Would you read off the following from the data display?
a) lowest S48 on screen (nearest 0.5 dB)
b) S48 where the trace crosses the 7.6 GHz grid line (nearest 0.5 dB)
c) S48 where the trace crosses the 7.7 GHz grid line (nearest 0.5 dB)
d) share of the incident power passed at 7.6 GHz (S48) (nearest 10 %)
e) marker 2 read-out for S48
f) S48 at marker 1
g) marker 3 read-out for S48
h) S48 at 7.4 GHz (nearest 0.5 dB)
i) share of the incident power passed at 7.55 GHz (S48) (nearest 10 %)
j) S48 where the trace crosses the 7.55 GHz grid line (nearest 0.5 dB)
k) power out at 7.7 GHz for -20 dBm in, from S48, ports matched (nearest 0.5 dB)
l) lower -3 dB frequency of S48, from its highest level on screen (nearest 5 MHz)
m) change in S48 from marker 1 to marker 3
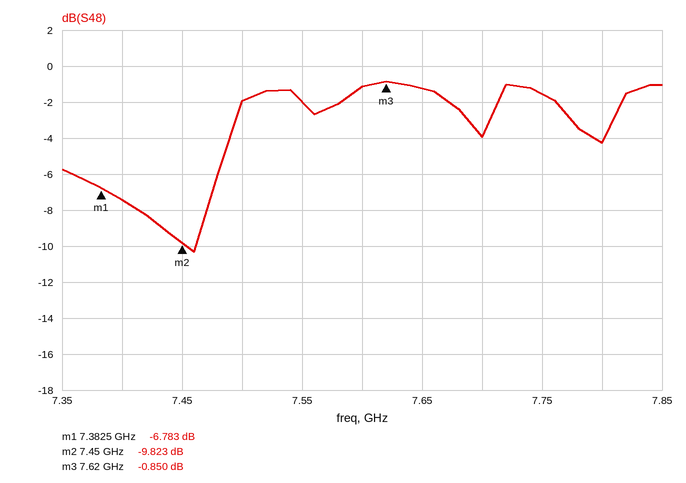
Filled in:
-10.5 dB
-1.0 dB
-4.0 dB
80 %
-9.823 dB
-6.783 dB
-0.850 dB
-7.5 dB
60 %
-2.0 dB
-24.0 dBm
7.490 GHz
5.933 dB
